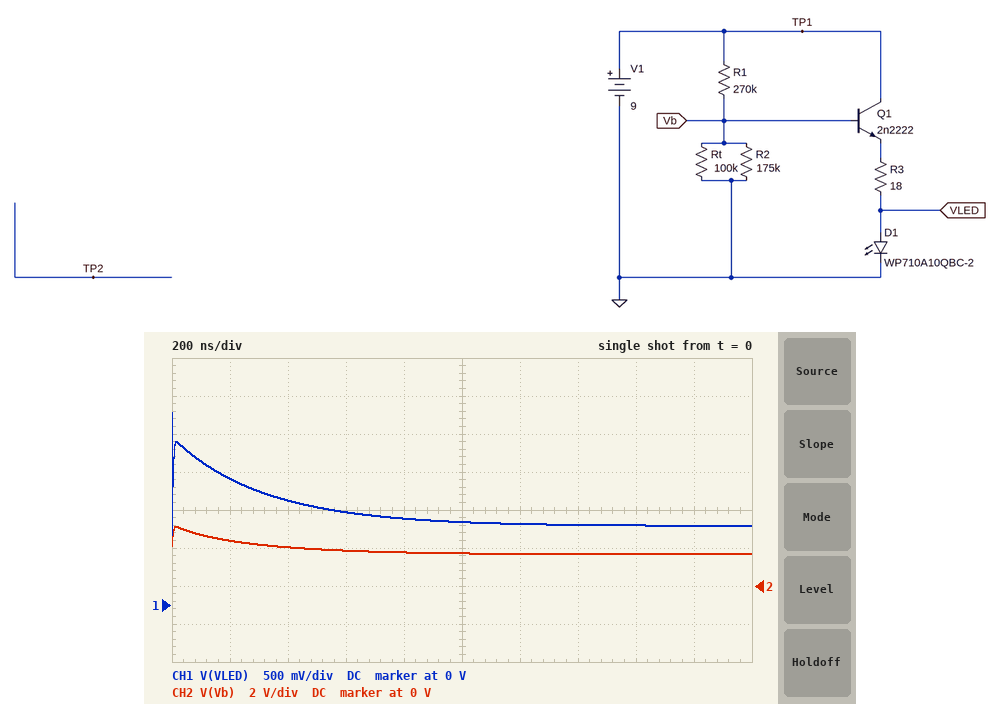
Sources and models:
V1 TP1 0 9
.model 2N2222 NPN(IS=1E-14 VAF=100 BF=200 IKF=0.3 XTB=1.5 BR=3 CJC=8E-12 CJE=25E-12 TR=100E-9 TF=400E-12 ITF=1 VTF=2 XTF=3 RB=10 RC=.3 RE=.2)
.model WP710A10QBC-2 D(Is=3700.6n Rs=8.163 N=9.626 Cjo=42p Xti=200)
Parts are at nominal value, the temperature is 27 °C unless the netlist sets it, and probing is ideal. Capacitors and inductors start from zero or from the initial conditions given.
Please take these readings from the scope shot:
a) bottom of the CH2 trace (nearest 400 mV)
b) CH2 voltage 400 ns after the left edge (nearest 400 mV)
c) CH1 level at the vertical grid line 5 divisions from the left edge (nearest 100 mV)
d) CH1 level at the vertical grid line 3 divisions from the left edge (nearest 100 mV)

1.6 V
2.0 V
1.1 V
1.2 V
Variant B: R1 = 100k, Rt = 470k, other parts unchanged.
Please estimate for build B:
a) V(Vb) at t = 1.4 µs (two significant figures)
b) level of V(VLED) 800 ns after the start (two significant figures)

2.8 V
2.0 V
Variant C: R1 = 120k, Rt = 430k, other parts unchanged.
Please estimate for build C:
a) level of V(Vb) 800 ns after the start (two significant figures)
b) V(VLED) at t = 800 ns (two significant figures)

2.7 V
1.9 V
